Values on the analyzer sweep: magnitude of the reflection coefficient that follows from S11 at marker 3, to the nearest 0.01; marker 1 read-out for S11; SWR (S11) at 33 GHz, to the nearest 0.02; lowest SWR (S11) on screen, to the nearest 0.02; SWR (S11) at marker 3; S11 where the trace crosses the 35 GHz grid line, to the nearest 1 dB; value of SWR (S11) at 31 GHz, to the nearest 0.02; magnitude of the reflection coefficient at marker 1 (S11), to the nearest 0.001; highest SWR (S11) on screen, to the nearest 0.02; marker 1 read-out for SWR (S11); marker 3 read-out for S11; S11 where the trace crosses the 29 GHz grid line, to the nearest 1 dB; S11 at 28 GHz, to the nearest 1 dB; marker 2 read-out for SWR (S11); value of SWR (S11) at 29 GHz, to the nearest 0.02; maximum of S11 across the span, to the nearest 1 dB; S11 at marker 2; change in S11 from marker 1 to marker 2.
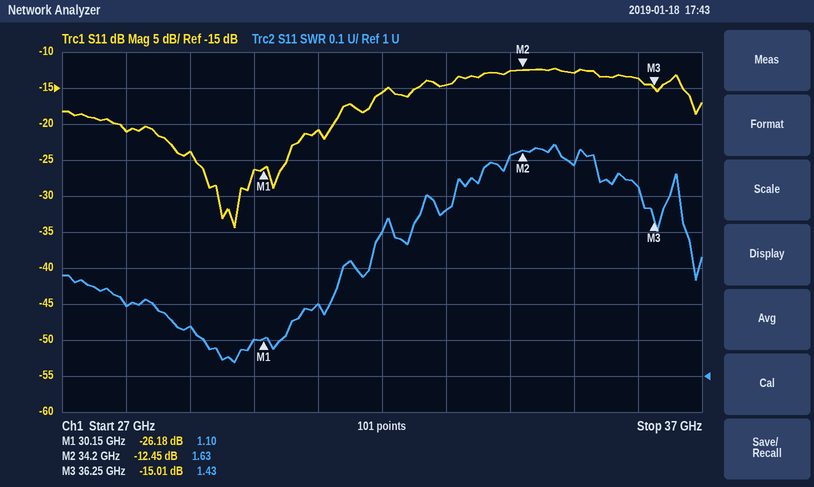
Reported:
0.18
-26.18 dB
1.46
1.04
1.43
-13 dB
1.20
0.049
1.64
1.10
-15.01 dB
-24 dB
-21 dB
1.63
1.14
-12 dB
-12.45 dB
13.73 dB
